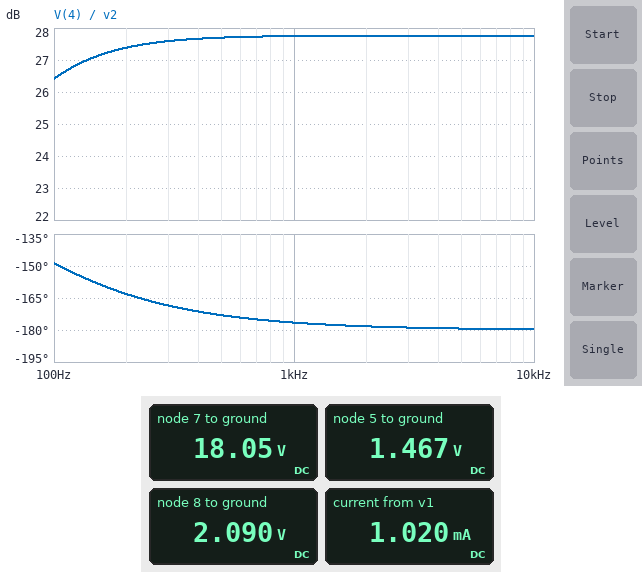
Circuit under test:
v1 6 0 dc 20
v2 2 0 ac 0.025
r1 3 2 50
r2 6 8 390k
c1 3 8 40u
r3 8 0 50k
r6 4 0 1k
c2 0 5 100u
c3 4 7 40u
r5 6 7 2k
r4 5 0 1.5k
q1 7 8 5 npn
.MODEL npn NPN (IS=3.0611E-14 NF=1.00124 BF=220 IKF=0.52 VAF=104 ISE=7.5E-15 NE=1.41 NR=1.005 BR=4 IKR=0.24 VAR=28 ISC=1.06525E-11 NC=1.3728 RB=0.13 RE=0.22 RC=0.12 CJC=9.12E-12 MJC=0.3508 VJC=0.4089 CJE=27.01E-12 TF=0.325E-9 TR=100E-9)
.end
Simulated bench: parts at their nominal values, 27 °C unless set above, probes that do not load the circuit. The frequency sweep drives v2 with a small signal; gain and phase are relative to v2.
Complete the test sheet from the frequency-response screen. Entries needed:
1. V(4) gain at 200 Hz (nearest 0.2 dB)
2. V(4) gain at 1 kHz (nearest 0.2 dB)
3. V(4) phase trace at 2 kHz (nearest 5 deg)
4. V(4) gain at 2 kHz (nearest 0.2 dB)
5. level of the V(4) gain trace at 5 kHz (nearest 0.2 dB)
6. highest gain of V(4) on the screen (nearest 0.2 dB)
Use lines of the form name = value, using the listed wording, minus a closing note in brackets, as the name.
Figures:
V(4) gain at 200 Hz = 27.4 dB
V(4) gain at 1 kHz = 27.8 dB
V(4) phase trace at 2 kHz = -180 deg
V(4) gain at 2 kHz = 27.8 dB
level of the V(4) gain trace at 5 kHz = 27.8 dB
highest gain of V(4) on the screen = 27.8 dB
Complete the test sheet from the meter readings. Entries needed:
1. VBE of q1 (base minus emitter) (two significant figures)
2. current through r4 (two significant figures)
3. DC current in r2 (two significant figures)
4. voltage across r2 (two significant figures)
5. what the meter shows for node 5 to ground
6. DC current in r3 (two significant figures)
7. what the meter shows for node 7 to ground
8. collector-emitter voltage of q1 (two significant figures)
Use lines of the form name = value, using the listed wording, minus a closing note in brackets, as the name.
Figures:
VBE of q1 (base minus emitter) = 620 mV
current through r4 = 980 µA
DC current in r2 = 46 µA
voltage across r2 = 18 V
what the meter shows for node 5 to ground = 1.467 V
DC current in r3 = 42 µA
what the meter shows for node 7 to ground = 18.05 V
collector-emitter voltage of q1 = 17 V
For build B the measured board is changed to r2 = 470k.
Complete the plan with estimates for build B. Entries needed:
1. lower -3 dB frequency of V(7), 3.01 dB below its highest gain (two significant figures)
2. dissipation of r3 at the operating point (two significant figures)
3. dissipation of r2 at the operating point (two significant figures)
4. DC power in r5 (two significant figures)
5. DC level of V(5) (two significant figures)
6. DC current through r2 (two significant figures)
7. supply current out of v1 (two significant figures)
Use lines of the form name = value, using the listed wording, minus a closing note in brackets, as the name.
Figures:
lower -3 dB frequency of V(7), 3.01 dB below its highest gain = 48 Hz
dissipation of r3 at the operating point = 63 µW
dissipation of r2 at the operating point = 710 µW
DC power in r5 = 1.2 mW
DC level of V(5) = 1.2 V
DC current through r2 = 39 µA
supply current out of v1 = 810 µA
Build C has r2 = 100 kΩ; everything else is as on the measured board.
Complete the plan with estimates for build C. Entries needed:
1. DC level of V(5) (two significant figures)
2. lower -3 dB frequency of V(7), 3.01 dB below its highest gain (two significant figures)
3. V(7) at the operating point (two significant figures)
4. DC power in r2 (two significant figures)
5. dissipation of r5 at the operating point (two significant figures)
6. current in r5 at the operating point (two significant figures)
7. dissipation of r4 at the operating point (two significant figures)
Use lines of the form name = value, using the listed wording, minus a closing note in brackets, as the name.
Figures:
DC level of V(5) = 5.5 V
lower -3 dB frequency of V(7), 3.01 dB below its highest gain = 210 Hz
V(7) at the operating point = 13 V
DC power in r2 = 1.9 mW
dissipation of r5 at the operating point = 26 mW
current in r5 at the operating point = 3.6 mA
dissipation of r4 at the operating point = 20 mW
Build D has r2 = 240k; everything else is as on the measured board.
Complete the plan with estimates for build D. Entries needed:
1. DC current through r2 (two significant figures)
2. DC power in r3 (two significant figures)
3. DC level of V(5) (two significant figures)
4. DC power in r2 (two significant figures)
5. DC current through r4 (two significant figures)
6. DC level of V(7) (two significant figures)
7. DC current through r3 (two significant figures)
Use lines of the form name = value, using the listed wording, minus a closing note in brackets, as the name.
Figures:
DC current through r2 = 70 µA
DC power in r3 = 200 µW
DC level of V(5) = 2.5 V
DC power in r2 = 1.2 mW
DC current through r4 = 1.7 mA
DC level of V(7) = 17 V
DC current through r3 = 63 µA
